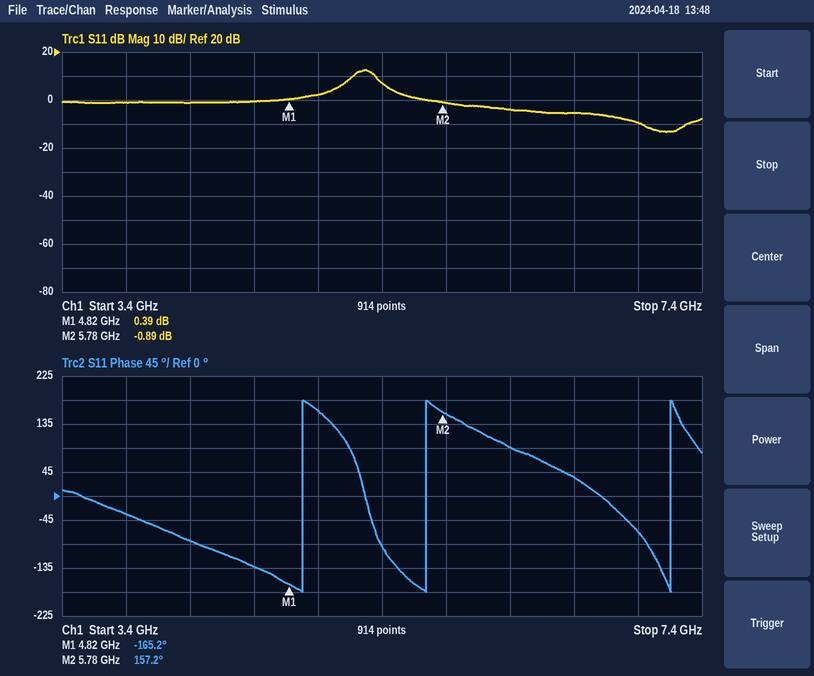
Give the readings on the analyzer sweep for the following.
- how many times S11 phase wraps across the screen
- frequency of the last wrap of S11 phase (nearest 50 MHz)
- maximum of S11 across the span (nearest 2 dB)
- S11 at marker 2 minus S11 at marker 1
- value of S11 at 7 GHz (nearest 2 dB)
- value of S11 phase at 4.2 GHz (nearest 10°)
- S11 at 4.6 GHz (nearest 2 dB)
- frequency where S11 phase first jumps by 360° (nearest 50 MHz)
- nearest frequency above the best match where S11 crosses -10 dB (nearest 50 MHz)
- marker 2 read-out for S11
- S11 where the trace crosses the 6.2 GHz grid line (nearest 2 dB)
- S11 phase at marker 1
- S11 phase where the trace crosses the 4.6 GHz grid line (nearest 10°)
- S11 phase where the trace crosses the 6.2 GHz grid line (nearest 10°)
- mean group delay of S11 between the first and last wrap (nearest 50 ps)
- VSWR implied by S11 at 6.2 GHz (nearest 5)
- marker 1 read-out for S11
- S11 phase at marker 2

3
7.20 GHz
12 dB
-1.28 dB
-10 dB
-80°
0 dB
4.90 GHz
7.30 GHz
-0.89 dB
-4 dB
-165.2°
-130°
90°
850 ps
5
0.39 dB
157.2°
